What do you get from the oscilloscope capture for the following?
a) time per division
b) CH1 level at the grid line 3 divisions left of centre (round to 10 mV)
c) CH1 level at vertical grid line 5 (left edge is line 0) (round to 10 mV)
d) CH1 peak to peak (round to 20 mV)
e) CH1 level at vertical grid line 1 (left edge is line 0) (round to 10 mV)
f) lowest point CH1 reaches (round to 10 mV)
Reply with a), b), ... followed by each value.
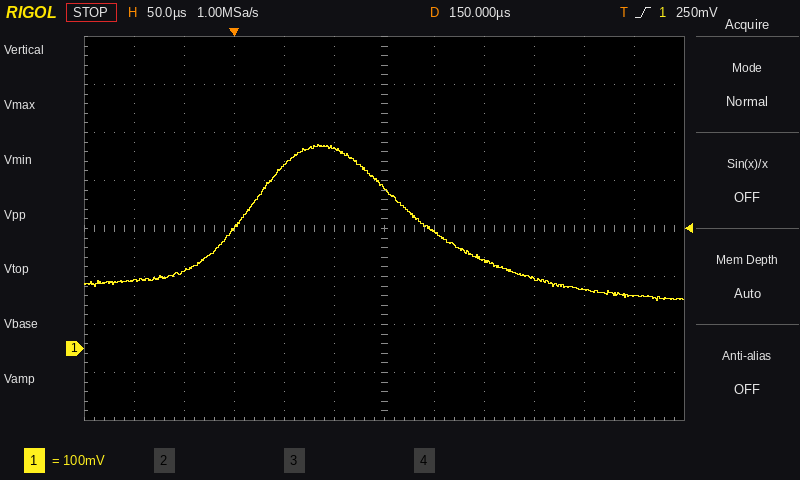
a) 50 µs
b) 250 mV
c) 420 mV
d) 320 mV
e) 140 mV
f) 100 mV
